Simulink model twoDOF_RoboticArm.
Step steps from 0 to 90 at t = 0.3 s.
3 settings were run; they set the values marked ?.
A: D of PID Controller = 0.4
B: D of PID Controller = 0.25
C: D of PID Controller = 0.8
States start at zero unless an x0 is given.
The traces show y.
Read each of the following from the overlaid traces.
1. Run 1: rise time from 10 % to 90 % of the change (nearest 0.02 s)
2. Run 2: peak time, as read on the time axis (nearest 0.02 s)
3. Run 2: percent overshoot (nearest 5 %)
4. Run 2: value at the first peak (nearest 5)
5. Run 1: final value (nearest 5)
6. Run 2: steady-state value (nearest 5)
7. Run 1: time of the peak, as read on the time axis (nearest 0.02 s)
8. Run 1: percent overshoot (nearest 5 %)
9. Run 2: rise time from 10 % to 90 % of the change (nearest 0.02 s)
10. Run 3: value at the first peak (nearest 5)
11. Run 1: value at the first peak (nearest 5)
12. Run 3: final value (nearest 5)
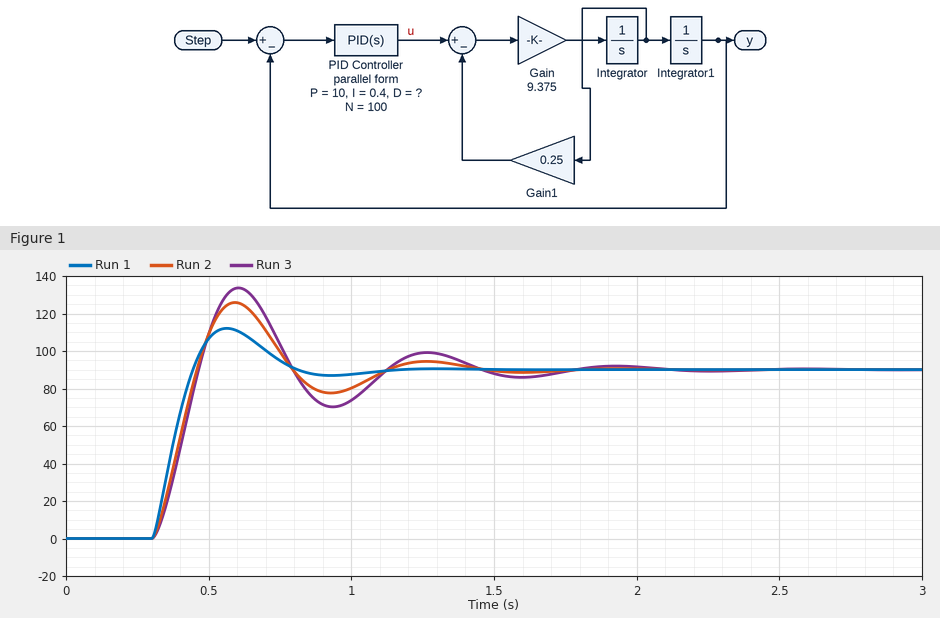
0.10 s
0.60 s
40 %
125
90
90
0.56 s
25 %
0.12 s
135
110
90
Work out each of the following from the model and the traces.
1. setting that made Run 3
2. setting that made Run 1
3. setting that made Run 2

B
C
A
